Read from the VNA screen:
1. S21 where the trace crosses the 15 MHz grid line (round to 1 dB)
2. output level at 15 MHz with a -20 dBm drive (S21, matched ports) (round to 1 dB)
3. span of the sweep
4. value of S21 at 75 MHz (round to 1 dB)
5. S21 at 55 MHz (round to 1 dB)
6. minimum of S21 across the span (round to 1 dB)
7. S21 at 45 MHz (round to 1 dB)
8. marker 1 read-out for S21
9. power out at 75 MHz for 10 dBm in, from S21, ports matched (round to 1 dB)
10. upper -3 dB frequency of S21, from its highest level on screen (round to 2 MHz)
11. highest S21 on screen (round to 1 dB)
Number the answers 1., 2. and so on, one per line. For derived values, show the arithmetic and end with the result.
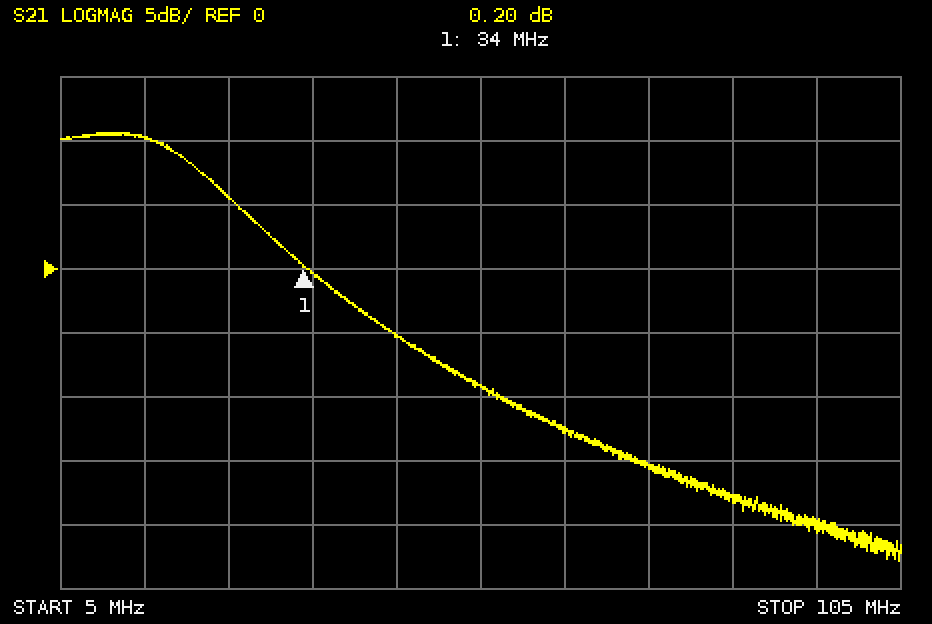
1. 10 dB
2. -20 dBm + (10 dB) = -10 dBm
3. 100 MHz
4. -15 dB
5. -9 dB
6. -23 dB
7. -5 dB
8. 0.20 dB
9. 10 dBm + (-15 dB) = -5 dBm
10. 22 MHz
11. 11 dB
